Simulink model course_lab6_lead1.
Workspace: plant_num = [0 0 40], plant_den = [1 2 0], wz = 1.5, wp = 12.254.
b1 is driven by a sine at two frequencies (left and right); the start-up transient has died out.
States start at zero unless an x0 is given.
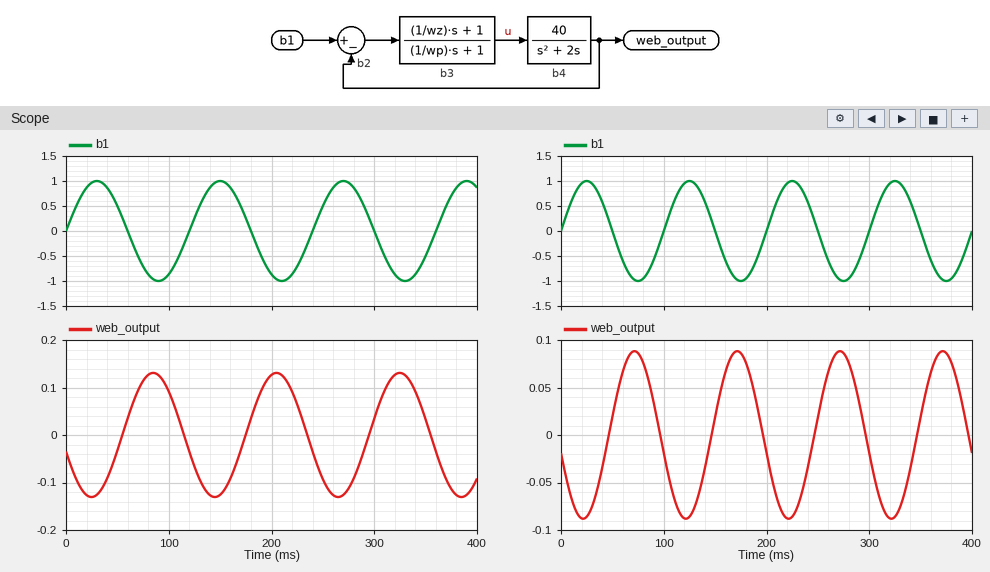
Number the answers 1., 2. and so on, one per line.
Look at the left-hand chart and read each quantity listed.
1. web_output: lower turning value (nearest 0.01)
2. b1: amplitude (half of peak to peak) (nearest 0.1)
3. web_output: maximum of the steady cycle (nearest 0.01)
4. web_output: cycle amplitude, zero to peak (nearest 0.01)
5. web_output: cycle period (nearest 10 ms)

1. -0.13
2. 1.0
3. 0.13
4. 0.13
5. 120 ms
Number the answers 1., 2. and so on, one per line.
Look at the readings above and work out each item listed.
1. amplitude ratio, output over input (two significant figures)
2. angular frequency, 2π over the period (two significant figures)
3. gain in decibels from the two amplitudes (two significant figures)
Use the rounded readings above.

1. 0.13
2. 0.052 rad/ms
3. -18 dB
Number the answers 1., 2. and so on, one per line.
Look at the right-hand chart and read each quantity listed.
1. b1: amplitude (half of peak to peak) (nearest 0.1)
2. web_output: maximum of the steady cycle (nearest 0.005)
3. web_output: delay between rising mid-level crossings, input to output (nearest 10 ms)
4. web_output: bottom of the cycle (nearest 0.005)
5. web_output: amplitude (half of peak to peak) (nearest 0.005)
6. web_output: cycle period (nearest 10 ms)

1. 1.0
2. 0.090
3. 50 ms
4. -0.090
5. 0.090
6. 100 ms
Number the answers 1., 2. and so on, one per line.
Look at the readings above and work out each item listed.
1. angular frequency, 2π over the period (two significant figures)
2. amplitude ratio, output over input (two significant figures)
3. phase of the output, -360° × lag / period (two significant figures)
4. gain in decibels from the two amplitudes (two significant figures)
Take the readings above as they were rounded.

1. 0.063 rad/ms
2. 0.090
3. -180°
4. -21 dB
